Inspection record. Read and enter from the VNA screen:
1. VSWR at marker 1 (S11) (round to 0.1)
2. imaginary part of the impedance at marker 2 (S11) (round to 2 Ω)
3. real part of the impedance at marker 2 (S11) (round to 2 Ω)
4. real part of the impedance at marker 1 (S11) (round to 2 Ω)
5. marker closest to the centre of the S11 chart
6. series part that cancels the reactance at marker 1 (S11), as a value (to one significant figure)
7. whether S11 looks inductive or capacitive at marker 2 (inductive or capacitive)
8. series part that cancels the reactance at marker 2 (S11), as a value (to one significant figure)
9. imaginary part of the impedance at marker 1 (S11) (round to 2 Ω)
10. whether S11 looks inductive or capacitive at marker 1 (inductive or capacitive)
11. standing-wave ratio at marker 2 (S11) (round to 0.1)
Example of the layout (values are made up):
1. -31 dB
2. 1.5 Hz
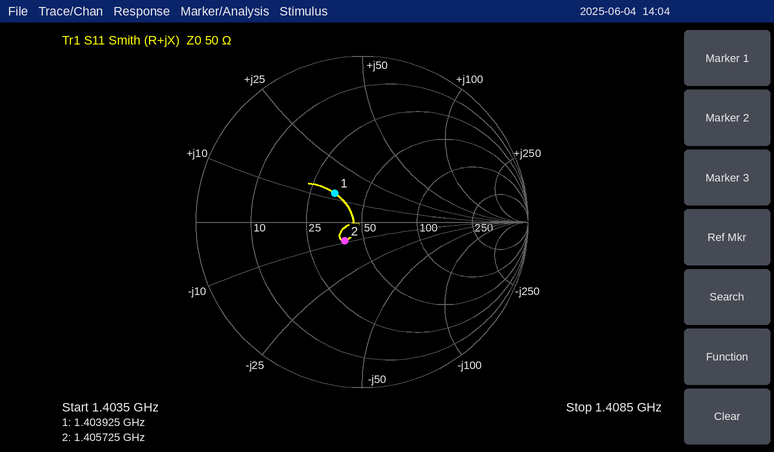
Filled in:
1. 1.6
2. -10 Ω
3. 40 Ω
4. 34 Ω
5. marker 2
6. 9 pF
7. capacitive
8. 1 nH
9. +12 Ω
10. inductive
11. 1.4
